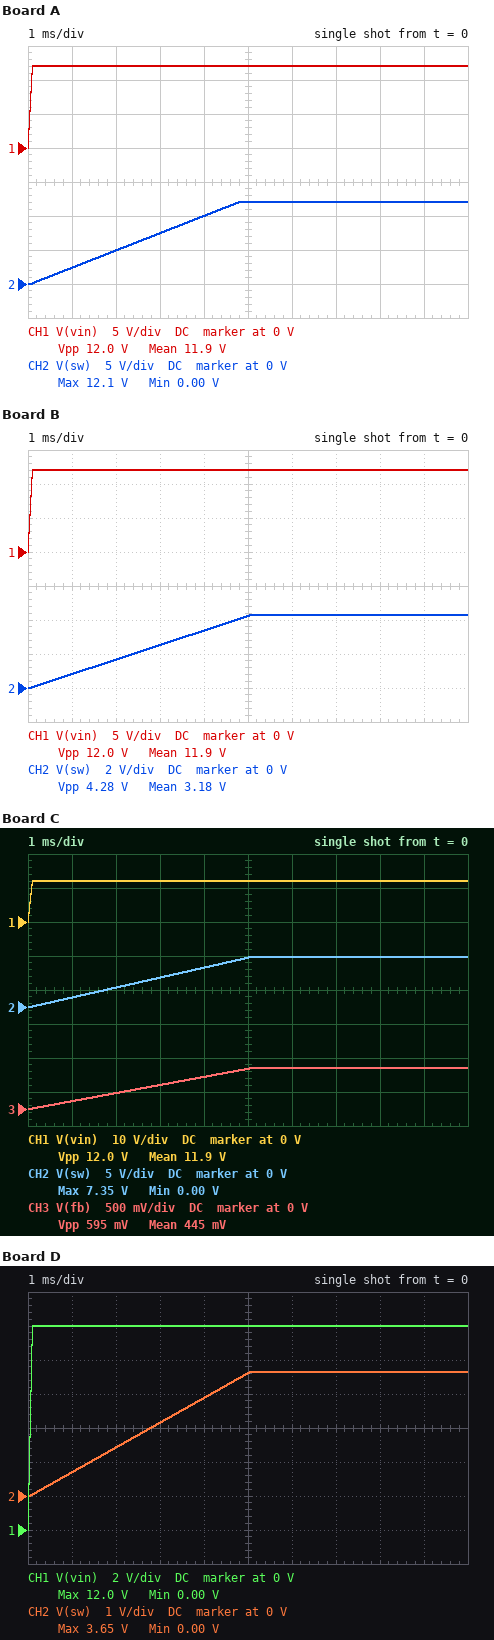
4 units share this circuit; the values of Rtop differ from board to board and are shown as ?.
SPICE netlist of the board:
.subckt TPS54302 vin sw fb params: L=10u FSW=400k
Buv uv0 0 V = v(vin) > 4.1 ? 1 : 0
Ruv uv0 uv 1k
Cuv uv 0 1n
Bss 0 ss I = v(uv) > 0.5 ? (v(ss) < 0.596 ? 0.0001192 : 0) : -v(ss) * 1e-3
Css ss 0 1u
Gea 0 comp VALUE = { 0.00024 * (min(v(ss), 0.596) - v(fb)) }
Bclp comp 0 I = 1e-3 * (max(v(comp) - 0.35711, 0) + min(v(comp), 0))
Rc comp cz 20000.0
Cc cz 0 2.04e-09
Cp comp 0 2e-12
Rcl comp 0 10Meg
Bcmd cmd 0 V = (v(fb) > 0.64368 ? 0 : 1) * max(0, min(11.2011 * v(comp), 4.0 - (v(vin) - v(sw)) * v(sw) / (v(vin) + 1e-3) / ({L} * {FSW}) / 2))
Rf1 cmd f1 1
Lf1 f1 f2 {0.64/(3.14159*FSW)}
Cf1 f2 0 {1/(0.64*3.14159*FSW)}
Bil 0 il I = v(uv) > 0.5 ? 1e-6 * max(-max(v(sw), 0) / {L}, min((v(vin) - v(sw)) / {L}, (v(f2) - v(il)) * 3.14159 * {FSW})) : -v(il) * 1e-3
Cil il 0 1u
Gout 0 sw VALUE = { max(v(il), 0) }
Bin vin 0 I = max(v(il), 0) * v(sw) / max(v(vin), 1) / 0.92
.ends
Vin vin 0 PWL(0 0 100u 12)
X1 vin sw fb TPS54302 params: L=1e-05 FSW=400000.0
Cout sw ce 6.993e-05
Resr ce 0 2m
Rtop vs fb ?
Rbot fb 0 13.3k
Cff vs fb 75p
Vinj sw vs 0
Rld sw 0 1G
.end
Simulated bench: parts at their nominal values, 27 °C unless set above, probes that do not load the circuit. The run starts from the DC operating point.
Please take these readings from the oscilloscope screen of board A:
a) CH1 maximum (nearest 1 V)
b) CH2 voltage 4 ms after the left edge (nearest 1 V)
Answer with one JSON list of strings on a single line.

["12 V", "10 V"]
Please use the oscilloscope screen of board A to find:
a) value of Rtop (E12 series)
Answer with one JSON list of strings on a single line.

["270 kΩ"]
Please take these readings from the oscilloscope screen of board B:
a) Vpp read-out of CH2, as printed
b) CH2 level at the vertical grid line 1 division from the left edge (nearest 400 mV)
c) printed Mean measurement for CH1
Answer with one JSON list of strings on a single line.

["4.28 V", "800 mV", "11.9 V"]
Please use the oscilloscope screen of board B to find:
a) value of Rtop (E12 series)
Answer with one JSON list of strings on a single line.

["82 kΩ"]
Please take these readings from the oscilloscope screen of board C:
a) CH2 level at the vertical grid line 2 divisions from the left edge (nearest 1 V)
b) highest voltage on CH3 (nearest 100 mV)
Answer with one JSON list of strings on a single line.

["3 V", "600 mV"]
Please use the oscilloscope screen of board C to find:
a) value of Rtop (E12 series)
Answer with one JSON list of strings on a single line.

["150 kΩ"]
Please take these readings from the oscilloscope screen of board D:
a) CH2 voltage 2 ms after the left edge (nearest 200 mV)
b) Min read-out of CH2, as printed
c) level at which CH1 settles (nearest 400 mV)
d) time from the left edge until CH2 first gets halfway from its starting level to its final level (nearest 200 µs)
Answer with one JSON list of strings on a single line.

["1.4 V", "0.00 V", "12.0 V", "2.6 ms"]
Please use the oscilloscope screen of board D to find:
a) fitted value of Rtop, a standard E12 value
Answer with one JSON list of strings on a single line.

["68 kΩ"]
